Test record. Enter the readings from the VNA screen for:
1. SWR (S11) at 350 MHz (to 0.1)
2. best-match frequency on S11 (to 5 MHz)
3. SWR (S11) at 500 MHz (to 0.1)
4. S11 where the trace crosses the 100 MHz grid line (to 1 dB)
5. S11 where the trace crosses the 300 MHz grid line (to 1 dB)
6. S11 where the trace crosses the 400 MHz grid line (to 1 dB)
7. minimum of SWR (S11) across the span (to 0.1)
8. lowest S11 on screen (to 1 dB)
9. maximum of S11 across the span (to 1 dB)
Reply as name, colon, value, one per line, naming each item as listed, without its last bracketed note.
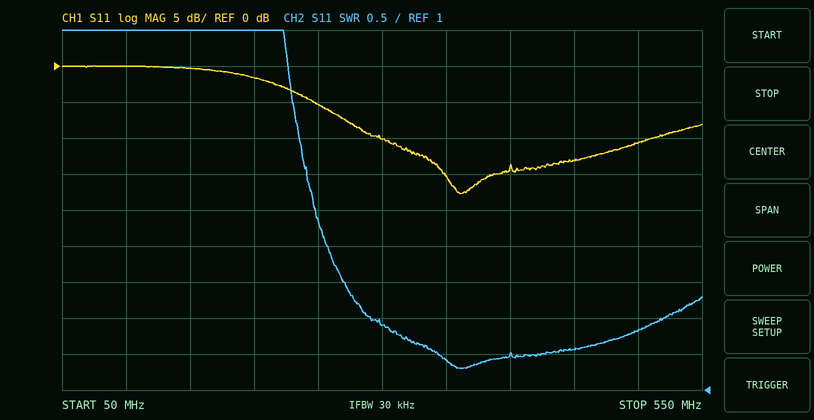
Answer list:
SWR (S11) at 350 MHz: 1.4
best-match frequency on S11: 360 MHz
SWR (S11) at 500 MHz: 1.8
S11 where the trace crosses the 100 MHz grid line: 0 dB
S11 where the trace crosses the 300 MHz grid line: -10 dB
S11 where the trace crosses the 400 MHz grid line: -14 dB
minimum of SWR (S11) across the span: 1.3
lowest S11 on screen: -18 dB
maximum of S11 across the span: 0 dB
